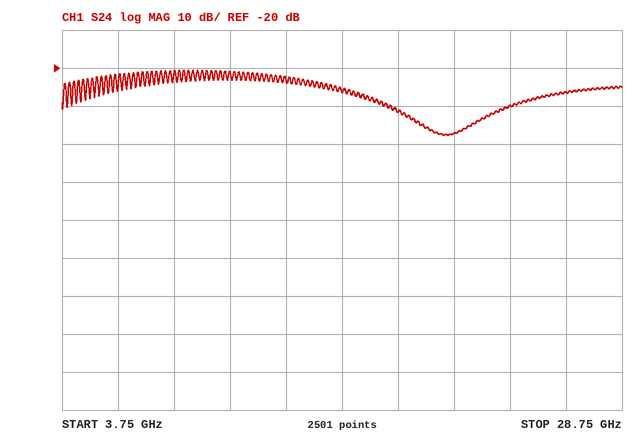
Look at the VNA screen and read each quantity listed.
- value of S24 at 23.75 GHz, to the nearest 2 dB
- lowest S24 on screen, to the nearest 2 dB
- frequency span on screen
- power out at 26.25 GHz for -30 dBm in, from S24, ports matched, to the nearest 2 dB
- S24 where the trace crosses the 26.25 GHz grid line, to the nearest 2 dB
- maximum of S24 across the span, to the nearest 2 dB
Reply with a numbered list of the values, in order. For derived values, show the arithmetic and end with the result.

1. -30 dB
2. -38 dB
3. 25 GHz
4. -30 dBm + (-26 dB) = -56 dBm
5. -26 dB
6. -20 dB
